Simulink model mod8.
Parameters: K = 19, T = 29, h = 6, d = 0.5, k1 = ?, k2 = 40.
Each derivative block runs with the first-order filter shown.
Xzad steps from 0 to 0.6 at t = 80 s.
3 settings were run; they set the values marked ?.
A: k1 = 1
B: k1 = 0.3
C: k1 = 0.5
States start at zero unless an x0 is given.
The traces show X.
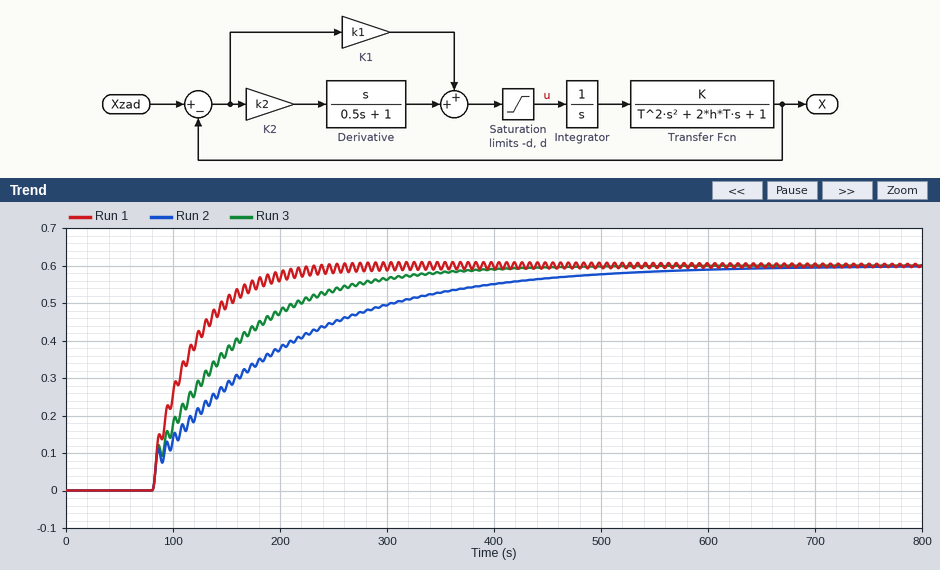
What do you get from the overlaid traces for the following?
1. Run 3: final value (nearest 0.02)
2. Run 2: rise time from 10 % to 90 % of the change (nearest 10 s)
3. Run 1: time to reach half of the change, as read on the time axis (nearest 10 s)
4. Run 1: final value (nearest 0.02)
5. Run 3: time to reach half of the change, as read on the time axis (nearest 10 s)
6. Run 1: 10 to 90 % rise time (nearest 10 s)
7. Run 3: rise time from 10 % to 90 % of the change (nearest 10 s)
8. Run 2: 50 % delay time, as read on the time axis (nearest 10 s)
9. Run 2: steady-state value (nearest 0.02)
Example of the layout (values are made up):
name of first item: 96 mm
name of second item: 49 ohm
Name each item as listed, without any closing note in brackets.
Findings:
Run 3: final value: 0.60
Run 2: rise time from 10 % to 90 % of the change: 290 s
Run 1: time to reach half of the change, as read on the time axis: 110 s
Run 1: final value: 0.60
Run 3: time to reach half of the change, as read on the time axis: 130 s
Run 1: 10 to 90 % rise time: 80 s
Run 3: rise time from 10 % to 90 % of the change: 170 s
Run 2: 50 % delay time, as read on the time axis: 160 s
Run 2: steady-state value: 0.60
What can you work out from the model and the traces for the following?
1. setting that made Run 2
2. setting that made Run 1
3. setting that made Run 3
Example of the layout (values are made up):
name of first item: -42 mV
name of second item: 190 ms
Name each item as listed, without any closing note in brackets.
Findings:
setting that made Run 2: B
setting that made Run 1: A
setting that made Run 3: C
